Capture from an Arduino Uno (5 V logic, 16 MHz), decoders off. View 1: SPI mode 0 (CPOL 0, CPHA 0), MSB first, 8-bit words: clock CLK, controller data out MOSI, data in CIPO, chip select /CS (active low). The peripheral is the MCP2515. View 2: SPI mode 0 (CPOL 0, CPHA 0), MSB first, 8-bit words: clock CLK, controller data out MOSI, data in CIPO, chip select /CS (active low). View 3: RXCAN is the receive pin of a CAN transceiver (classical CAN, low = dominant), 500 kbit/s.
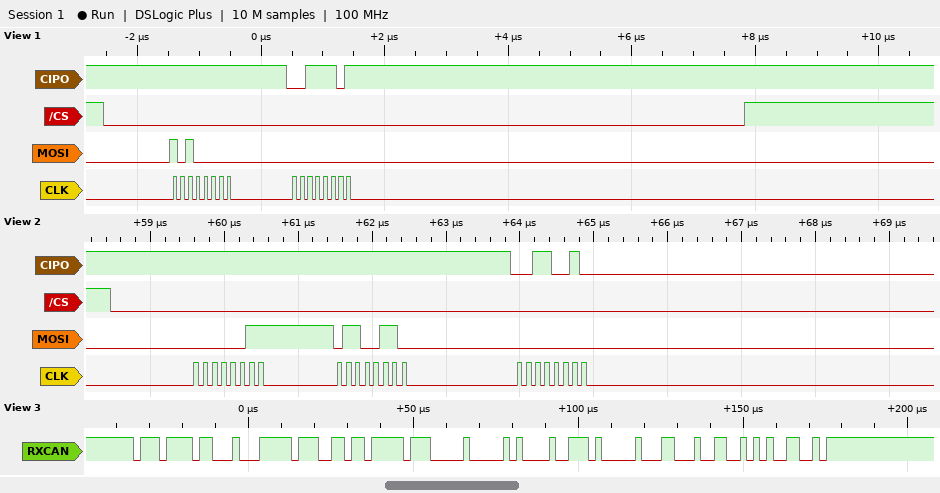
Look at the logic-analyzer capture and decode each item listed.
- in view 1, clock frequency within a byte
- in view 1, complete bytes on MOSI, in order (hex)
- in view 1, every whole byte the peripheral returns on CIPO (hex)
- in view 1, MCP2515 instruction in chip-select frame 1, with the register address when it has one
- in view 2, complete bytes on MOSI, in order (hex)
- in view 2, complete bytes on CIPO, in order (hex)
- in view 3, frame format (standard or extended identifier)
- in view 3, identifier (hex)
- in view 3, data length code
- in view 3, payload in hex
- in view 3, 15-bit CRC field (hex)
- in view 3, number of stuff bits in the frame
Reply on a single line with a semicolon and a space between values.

8 MHz; 0xA0 0x00; 0xFF 0x3D; READ STATUS; 03 66 00; FF FF 32; standard; 0x77B; 8; FF 36 FF 00 10 9D 00 C4; 0x654C; 5
